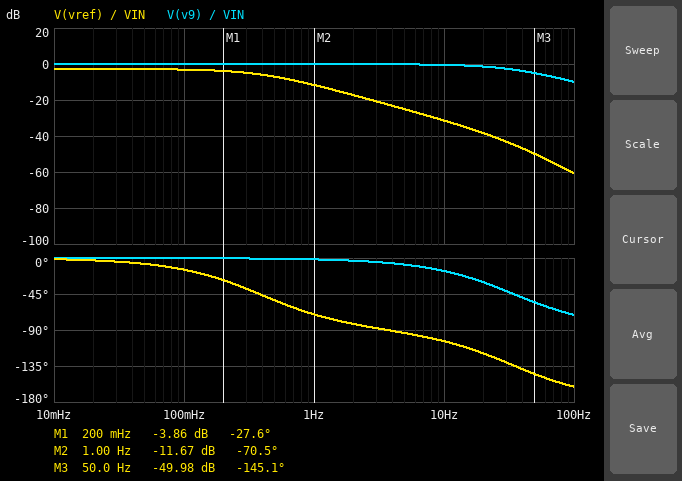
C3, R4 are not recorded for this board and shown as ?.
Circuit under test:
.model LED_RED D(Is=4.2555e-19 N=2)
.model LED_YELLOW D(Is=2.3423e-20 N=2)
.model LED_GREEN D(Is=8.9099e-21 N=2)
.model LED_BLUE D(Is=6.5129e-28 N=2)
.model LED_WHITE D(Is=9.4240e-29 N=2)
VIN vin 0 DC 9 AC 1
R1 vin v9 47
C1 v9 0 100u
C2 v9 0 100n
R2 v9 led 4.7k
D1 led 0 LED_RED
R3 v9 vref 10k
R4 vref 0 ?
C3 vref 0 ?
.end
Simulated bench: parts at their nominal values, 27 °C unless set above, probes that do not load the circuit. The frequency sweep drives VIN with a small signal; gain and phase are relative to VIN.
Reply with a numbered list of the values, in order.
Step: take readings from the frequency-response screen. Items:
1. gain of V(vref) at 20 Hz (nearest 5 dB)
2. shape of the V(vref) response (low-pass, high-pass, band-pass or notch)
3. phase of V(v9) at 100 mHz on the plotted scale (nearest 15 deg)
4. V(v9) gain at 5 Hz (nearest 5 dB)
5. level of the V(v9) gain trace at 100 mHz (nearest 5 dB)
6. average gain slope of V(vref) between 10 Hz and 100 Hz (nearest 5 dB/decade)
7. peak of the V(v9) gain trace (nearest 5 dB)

1. -40 dB
2. low-pass
3. 0 deg
4. 0 dB
5. 0 dB
6. -30 dB/decade
7. 0 dB
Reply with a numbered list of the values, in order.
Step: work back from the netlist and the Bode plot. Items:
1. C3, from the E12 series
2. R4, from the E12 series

1. 56 µF
2. 27 kΩ
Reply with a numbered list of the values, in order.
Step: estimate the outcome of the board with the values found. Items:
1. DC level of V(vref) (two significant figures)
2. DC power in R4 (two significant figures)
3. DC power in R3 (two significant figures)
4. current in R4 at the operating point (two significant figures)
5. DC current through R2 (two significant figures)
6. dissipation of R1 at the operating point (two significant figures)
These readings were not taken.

1. 6.5 V
2. 1.6 mW
3. 580 µW
4. 240 µA
5. 1.5 mA
6. 140 µW
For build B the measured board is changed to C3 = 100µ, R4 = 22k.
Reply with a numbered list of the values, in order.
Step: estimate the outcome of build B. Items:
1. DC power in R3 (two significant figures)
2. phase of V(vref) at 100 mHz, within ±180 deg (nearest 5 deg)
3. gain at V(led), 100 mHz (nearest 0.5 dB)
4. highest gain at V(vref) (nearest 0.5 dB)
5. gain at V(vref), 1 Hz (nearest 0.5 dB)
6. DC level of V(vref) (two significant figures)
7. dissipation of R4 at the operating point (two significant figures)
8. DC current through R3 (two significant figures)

1. 780 µW
2. -25 deg
3. -43.0 dB
4. -3.5 dB
5. -16.5 dB
6. 6.1 V
7. 1.7 mW
8. 280 µA
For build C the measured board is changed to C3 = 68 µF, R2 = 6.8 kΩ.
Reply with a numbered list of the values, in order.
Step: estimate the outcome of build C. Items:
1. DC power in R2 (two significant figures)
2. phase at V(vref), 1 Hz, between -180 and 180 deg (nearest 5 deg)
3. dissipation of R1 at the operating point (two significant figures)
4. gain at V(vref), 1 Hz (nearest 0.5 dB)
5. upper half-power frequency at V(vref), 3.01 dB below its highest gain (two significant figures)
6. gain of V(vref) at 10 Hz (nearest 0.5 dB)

1. 7.4 mW
2. -75 deg
3. 78 µW
4. -13.0 dB
5. 320 mHz
6. -33.0 dB
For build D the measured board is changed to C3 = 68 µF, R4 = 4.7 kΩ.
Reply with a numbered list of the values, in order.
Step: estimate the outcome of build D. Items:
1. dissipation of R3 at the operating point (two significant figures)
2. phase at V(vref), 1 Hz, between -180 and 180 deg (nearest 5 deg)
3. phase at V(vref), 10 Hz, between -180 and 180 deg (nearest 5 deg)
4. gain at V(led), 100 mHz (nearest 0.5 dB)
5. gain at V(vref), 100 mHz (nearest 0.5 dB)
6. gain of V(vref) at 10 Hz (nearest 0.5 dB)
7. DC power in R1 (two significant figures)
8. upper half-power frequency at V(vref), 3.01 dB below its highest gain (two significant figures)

1. 3.7 mW
2. -55 deg
3. -100 deg
4. -43.0 dB
5. -10.0 dB
6. -33.0 dB
7. 210 µW
8. 730 mHz
